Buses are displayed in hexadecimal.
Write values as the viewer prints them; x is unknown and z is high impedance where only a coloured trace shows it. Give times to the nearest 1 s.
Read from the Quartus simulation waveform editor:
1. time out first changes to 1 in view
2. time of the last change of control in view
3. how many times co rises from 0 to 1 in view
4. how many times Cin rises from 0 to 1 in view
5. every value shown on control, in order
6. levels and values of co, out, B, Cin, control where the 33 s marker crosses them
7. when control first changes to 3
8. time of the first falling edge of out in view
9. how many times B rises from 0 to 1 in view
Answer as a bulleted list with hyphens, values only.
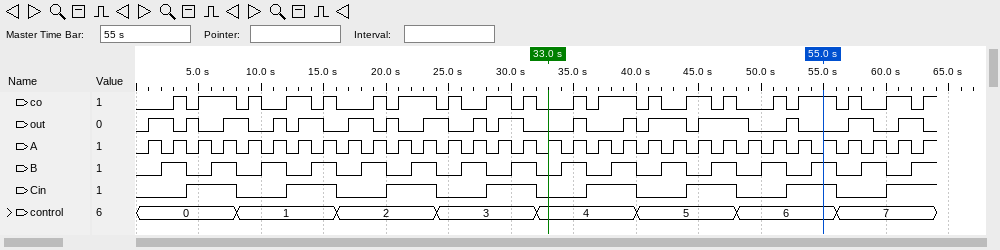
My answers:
- 1 s
- 56 s
- 20
- 8
- 0, 1, 2, 3, 4, 5, 6, 7
- co=0, out=0, B=0, Cin=0, control=4
- 24 s
- 3 s
- 16
